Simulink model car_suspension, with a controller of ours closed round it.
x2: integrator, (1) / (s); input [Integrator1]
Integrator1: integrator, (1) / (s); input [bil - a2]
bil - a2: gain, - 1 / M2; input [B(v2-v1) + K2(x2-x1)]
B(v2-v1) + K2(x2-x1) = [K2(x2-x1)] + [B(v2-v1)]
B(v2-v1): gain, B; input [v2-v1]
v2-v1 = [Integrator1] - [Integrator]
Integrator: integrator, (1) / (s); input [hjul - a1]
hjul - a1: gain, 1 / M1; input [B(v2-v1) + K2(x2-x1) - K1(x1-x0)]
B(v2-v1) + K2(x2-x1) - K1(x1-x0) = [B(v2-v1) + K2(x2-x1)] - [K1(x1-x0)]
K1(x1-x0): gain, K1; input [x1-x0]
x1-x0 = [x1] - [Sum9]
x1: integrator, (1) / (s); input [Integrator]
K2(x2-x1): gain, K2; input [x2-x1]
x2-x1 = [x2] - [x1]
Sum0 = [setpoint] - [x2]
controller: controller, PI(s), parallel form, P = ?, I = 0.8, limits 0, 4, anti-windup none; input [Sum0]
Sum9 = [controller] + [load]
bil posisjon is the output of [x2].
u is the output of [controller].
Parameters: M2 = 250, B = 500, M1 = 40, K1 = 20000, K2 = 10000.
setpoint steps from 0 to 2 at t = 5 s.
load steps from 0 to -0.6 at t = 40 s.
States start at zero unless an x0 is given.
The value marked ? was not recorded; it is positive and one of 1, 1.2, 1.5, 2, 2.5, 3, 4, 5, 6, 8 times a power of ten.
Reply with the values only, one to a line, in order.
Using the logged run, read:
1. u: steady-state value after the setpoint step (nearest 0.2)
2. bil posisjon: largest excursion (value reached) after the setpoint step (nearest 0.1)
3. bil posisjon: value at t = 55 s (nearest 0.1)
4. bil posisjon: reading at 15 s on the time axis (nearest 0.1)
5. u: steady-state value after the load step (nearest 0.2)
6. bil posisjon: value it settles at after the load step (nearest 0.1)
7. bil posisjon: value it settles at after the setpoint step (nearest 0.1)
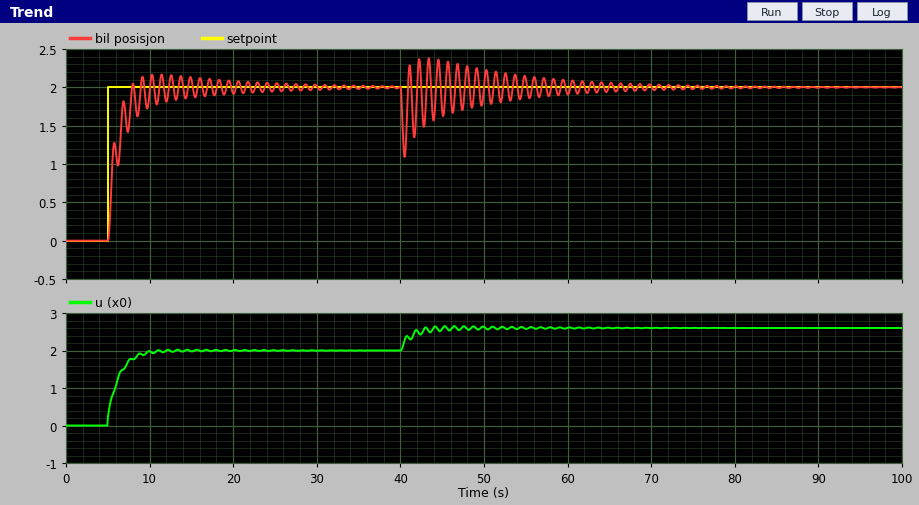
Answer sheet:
2.0
2.2
2.1
2.1
2.6
2.0
2.0
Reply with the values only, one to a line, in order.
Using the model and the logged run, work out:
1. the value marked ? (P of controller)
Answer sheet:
0.1
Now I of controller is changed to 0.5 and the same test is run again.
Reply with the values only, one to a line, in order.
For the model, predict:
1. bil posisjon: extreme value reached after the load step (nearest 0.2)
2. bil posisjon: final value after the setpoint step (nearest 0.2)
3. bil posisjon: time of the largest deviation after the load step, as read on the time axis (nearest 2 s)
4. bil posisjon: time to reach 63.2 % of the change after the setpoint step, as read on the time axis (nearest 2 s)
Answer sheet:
1.0
2.0
40 s
6 s
